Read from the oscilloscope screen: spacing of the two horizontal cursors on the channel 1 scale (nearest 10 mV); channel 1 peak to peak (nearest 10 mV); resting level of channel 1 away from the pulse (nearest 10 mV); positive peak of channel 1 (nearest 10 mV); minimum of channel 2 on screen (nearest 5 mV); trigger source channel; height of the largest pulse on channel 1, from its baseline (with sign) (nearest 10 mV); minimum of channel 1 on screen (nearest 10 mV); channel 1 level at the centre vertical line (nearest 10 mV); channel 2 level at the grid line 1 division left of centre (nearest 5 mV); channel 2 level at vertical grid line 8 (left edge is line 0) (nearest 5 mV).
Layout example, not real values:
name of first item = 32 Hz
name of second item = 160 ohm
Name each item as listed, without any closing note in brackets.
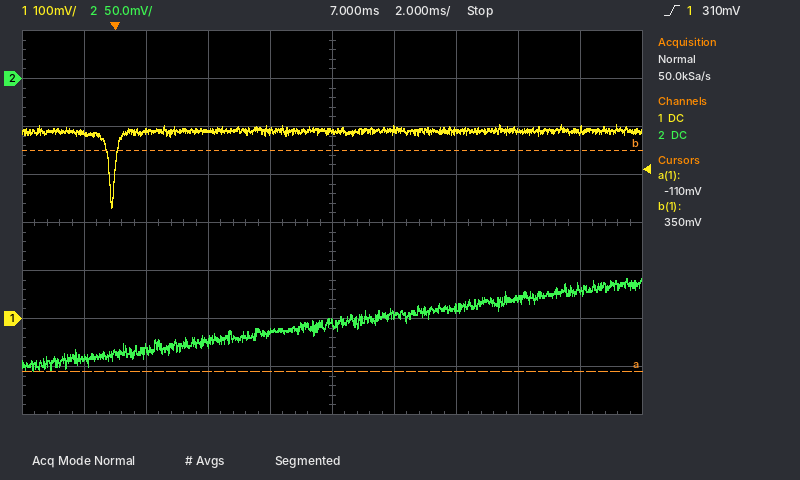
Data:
spacing of the two horizontal cursors on the channel 1 scale = 460 mV
channel 1 peak to peak = 170 mV
resting level of channel 1 away from the pulse = 390 mV
positive peak of channel 1 = 400 mV
minimum of channel 2 on screen = -305 mV
trigger source channel = channel 1
height of the largest pulse on channel 1, from its baseline (with sign) = -160 mV
minimum of channel 1 on screen = 230 mV
channel 1 level at the centre vertical line = 390 mV
channel 2 level at the grid line 1 division left of centre = -265 mV
channel 2 level at vertical grid line 8 (left edge is line 0) = -230 mV
